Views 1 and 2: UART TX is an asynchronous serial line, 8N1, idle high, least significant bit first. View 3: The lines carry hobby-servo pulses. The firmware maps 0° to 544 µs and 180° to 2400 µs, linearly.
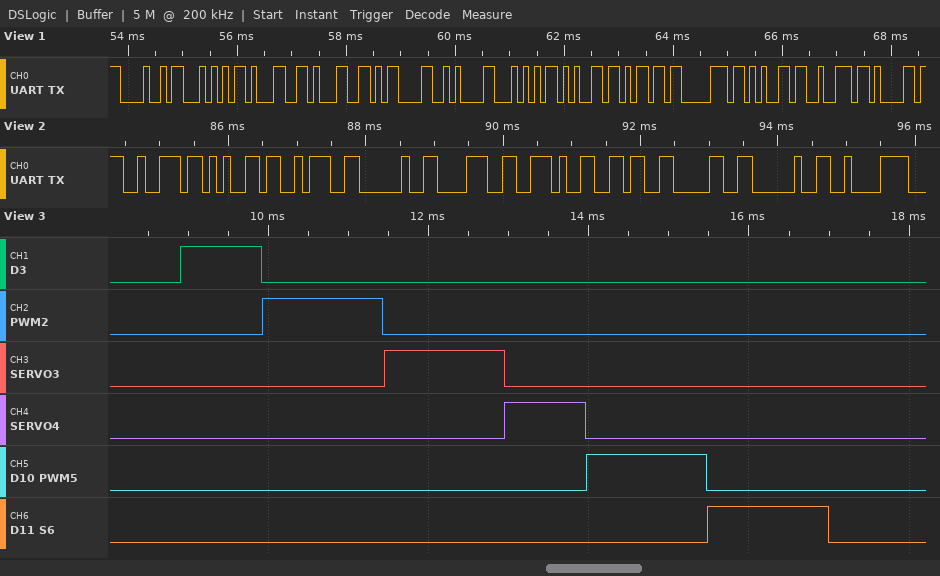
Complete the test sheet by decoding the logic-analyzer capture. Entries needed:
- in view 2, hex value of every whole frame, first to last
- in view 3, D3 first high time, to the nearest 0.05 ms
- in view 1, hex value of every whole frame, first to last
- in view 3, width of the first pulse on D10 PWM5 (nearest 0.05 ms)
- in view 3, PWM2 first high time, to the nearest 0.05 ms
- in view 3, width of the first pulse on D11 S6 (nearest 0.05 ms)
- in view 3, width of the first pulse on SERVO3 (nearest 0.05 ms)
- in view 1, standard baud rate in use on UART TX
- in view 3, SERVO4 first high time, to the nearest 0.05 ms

72 65 3A 20 38 2E 36 30 20 C2
1.00 ms
48 54 31 31 0D 0A 54 65 6D 70 65 72 61
1.50 ms
1.50 ms
1.50 ms
1.50 ms
9600 baud
1.00 ms
